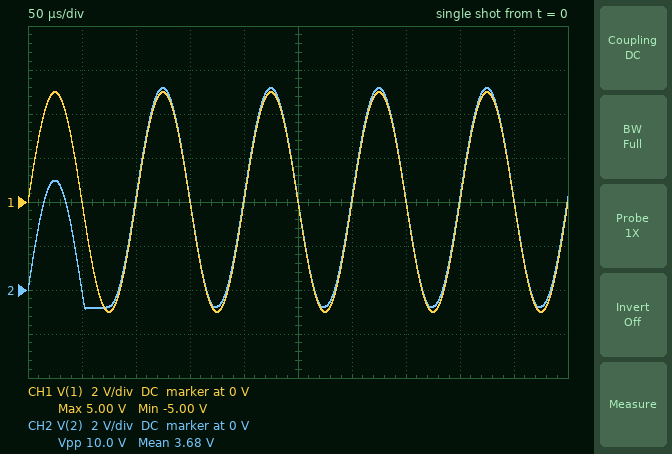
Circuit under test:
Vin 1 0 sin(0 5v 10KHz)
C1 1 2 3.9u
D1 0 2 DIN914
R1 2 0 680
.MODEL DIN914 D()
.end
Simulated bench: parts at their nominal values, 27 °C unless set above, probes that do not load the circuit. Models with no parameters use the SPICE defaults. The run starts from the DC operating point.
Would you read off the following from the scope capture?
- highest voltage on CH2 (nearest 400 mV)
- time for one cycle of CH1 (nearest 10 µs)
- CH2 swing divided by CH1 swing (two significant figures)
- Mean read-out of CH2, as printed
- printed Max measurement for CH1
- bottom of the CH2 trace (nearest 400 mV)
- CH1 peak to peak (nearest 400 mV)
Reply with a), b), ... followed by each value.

a) 9.2 V
b) 100 µs
c) 1.0
d) 3.68 V
e) 5.00 V
f) -800 mV
g) 10.0 V
